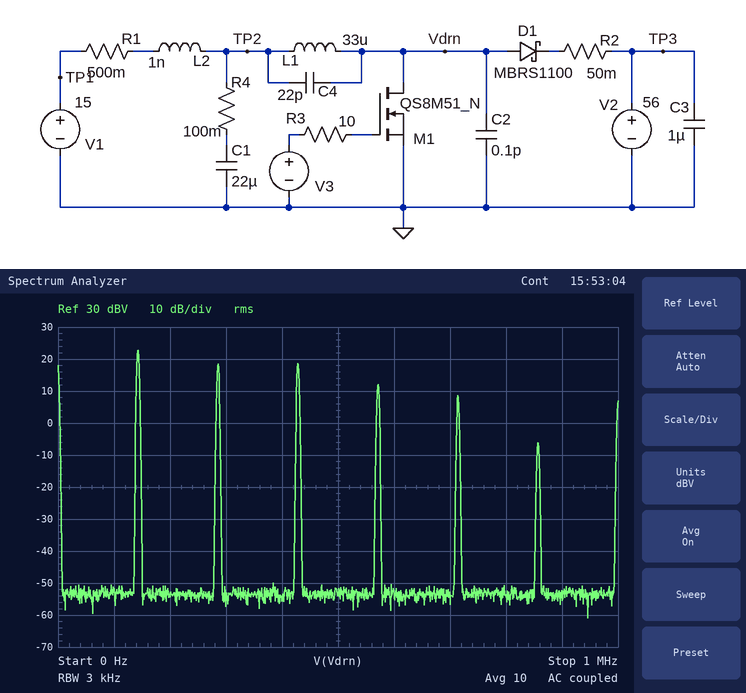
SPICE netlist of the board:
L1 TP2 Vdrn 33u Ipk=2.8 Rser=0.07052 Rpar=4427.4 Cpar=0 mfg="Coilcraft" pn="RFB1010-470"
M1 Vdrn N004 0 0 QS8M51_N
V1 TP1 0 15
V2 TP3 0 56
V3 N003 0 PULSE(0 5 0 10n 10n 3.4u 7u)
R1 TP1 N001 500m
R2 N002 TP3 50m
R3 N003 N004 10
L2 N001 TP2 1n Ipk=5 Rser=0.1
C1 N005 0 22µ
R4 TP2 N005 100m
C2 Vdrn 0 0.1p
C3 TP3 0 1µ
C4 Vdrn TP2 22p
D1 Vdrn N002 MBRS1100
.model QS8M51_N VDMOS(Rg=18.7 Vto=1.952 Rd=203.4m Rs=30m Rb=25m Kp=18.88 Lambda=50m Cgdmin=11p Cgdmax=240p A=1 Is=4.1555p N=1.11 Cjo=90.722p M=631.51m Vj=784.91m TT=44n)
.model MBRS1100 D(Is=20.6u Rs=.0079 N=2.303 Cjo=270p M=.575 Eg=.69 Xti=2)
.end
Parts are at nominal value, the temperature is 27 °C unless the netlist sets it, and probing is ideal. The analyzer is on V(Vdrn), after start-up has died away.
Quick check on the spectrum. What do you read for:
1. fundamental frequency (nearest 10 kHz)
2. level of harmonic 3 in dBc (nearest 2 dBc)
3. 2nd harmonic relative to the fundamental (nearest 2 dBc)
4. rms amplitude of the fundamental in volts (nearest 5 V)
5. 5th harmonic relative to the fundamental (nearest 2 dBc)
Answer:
140 kHz
-4 dBc
-4 dBc
15 V
-14 dBc
